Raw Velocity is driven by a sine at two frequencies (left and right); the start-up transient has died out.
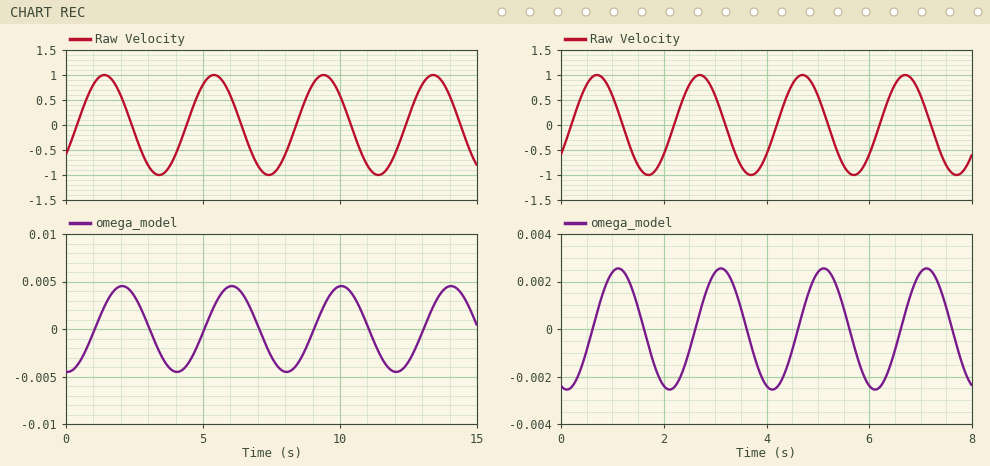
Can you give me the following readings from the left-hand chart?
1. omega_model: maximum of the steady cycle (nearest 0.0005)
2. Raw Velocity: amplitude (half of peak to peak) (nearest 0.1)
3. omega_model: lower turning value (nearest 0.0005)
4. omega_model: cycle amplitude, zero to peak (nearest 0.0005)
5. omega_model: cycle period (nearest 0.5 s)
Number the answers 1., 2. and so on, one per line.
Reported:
1. 0.0045
2. 1.0
3. -0.0045
4. 0.0045
5. 4.0 s
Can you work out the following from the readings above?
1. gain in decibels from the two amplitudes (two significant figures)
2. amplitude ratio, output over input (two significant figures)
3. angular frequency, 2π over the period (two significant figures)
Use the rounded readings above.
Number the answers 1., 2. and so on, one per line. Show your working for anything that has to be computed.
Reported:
1. 20 log10(0.0045 / 1) = -47 dB
2. 0.0045 / 1 = 0.0045
3. 2π / 4 = 1.6 rad/s
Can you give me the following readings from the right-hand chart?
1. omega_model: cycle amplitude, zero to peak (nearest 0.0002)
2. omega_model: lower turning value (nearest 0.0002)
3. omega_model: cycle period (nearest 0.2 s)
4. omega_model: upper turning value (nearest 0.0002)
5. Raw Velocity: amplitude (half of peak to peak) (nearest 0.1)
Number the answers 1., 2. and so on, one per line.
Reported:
1. 0.0026
2. -0.0026
3. 2.0 s
4. 0.0026
5. 1.0
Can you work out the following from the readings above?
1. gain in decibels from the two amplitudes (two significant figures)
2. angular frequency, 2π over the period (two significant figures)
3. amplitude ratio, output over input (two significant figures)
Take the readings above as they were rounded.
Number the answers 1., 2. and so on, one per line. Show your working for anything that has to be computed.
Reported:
1. 20 log10(0.0026 / 1) = -52 dB
2. 2π / 2 = 3.1 rad/s
3. 0.0026 / 1 = 0.0026
